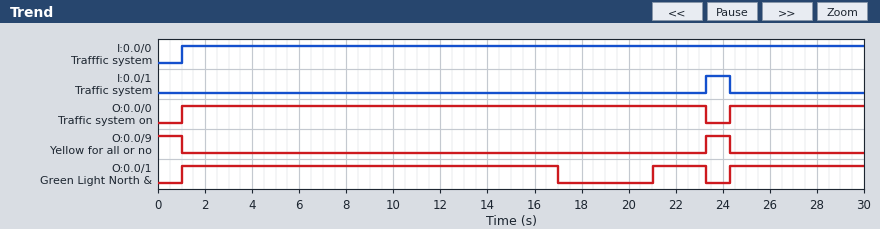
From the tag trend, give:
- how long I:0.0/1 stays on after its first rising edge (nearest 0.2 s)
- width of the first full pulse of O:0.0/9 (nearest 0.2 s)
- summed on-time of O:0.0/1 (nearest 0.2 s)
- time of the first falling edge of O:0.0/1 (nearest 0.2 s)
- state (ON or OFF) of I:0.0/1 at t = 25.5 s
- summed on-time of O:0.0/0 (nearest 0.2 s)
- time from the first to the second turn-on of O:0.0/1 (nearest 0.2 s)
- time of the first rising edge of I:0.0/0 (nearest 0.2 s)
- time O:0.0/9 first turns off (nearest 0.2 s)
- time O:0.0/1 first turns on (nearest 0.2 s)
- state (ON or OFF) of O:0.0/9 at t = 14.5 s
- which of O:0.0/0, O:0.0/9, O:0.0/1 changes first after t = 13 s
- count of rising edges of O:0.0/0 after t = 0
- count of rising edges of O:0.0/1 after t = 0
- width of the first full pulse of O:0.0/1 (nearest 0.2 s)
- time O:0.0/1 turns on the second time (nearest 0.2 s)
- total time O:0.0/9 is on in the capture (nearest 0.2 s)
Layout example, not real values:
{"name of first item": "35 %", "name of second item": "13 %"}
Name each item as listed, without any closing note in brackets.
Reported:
{"how long I:0.0/1 stays on after its first rising edge": "1.0 s", "width of the first full pulse of O:0.0/9": "1.0 s", "summed on-time of O:0.0/1": "24.0 s", "time of the first falling edge of O:0.0/1": "17.0 s", "state (ON or OFF) of I:0.0/1 at t = 25.5 s": "OFF", "summed on-time of O:0.0/0": "28.0 s", "time from the first to the second turn-on of O:0.0/1": "20.0 s", "time of the first rising edge of I:0.0/0": "1.0 s", "time O:0.0/9 first turns off": "1.0 s", "time O:0.0/1 first turns on": "1.0 s", "state (ON or OFF) of O:0.0/9 at t = 14.5 s": "OFF", "which of O:0.0/0, O:0.0/9, O:0.0/1 changes first after t = 13 s": "O:0.0/1", "count of rising edges of O:0.0/0 after t = 0": "2", "count of rising edges of O:0.0/1 after t = 0": "3", "width of the first full pulse of O:0.0/1": "16.0 s", "time O:0.0/1 turns on the second time": "21.0 s", "total time O:0.0/9 is on in the capture": "2.0 s"}
